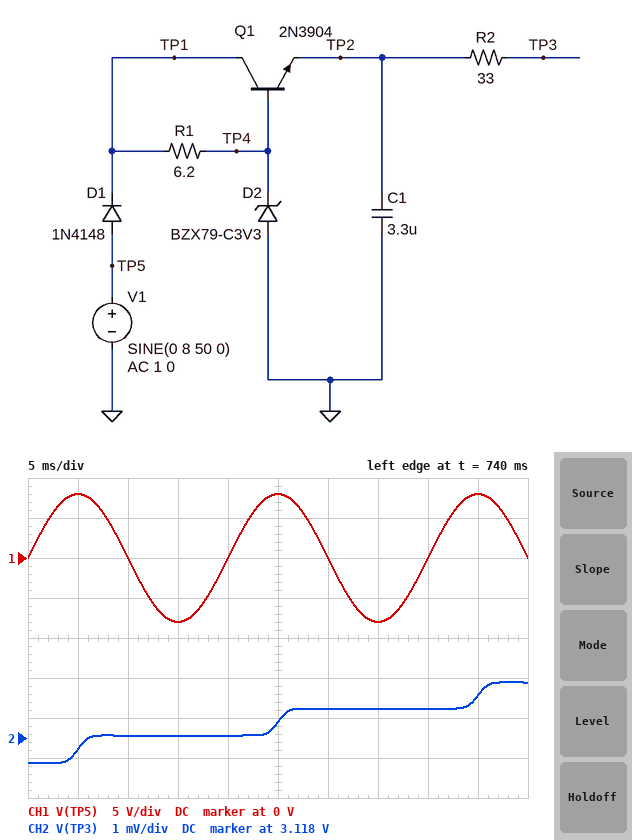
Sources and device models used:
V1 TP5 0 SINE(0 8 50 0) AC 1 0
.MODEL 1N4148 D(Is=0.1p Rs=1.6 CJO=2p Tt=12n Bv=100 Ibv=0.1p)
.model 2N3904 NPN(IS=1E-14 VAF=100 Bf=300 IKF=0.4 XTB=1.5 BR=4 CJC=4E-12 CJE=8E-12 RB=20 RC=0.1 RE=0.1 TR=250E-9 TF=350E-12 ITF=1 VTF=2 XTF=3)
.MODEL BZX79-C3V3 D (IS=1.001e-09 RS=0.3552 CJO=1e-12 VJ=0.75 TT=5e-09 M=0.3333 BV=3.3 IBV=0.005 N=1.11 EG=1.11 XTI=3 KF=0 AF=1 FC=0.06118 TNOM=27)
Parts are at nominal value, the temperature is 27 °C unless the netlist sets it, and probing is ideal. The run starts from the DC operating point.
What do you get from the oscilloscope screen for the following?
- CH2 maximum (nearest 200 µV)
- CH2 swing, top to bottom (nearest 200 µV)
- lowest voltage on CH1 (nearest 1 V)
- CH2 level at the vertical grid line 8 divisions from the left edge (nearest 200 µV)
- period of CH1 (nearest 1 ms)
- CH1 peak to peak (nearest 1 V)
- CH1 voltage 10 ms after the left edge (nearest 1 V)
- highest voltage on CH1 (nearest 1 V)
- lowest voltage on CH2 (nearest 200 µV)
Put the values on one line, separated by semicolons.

3.1194 V; 2.0 mV; -8 V; 3.1188 V; 20 ms; 16 V; 0 V; 8 V; 3.1174 V
